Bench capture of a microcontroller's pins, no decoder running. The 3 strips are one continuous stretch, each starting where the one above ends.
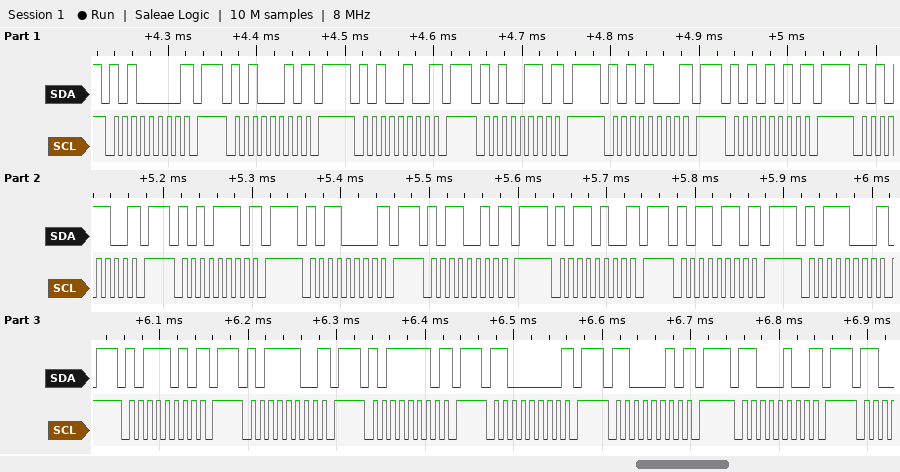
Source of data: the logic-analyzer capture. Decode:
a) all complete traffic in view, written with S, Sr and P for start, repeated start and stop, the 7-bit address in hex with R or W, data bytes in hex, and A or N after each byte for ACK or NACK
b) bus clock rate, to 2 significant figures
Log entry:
S 50W N P S 51W N P S 52W N P S 53W N P S 54W N P S 55W N P S 56W N P S 57W N P S 58W N P S 59W N P S 5AW N P S 5BW N P S 5CW N P S 5DW N P S 5EW N P S 5FW N P S 60W N P S 61W N P S 62W N P
100 kHz
